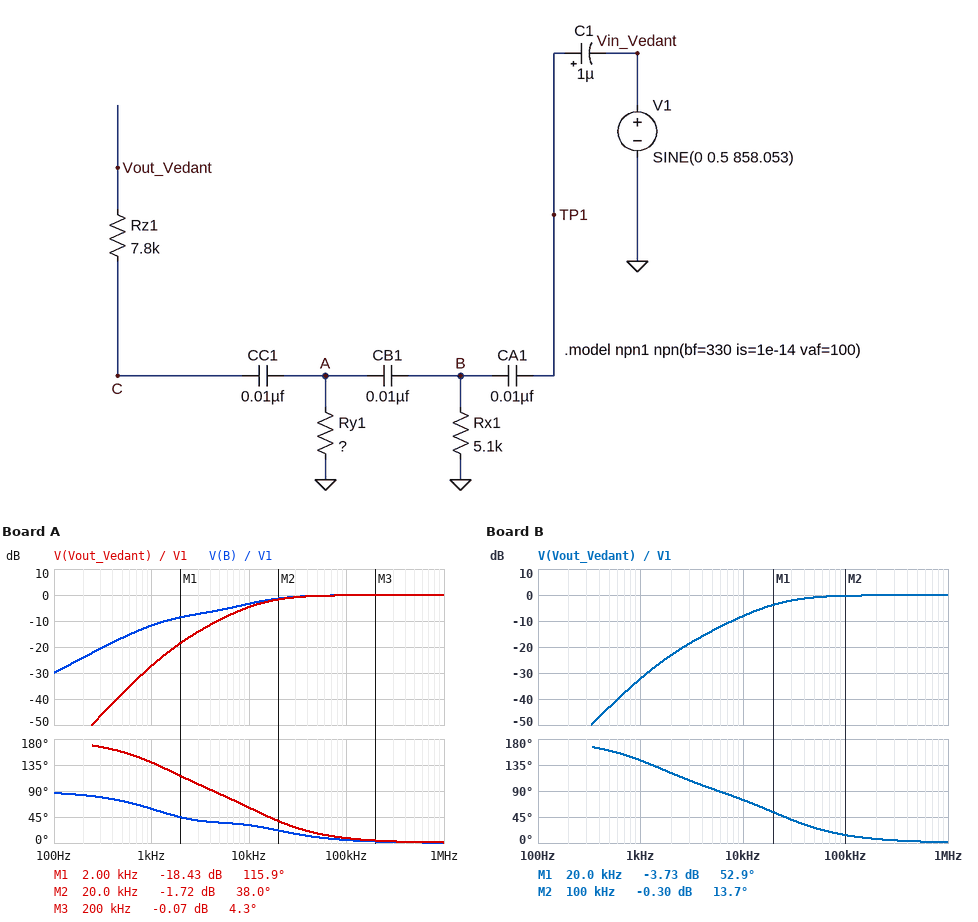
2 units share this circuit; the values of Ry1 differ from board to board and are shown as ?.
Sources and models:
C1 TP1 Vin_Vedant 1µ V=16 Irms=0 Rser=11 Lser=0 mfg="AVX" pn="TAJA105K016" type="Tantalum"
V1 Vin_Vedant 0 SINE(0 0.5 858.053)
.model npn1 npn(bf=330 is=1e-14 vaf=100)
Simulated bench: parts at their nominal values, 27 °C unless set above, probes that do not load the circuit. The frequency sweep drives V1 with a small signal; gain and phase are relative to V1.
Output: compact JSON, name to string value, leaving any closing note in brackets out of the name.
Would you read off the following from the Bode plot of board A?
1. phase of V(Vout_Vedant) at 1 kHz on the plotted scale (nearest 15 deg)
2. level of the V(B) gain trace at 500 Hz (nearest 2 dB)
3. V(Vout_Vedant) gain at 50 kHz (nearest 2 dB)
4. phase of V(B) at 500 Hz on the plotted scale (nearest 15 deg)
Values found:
{"phase of V(Vout_Vedant) at 1 kHz on the plotted scale": "135 deg", "level of the V(B) gain trace at 500 Hz": "-16 dB", "V(Vout_Vedant) gain at 50 kHz": "0 dB", "phase of V(B) at 500 Hz on the plotted scale": "75 deg"}
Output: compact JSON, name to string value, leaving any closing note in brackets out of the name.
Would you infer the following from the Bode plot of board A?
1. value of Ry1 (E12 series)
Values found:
{"value of Ry1": "2.7 kΩ"}
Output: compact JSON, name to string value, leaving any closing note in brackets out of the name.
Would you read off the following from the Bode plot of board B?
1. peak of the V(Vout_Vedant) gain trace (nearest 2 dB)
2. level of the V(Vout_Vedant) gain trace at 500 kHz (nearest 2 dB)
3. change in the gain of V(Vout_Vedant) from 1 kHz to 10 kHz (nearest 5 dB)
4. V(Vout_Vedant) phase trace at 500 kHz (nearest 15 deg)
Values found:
{"peak of the V(Vout_Vedant) gain trace": "0 dB", "level of the V(Vout_Vedant) gain trace at 500 kHz": "0 dB", "change in the gain of V(Vout_Vedant) from 1 kHz to 10 kHz": "25 dB", "V(Vout_Vedant) phase trace at 500 kHz": "0 deg"}
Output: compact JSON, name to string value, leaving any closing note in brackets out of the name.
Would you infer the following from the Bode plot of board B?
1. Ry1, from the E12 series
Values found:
{"Ry1, from the E12 series": "1.5 kΩ"}
